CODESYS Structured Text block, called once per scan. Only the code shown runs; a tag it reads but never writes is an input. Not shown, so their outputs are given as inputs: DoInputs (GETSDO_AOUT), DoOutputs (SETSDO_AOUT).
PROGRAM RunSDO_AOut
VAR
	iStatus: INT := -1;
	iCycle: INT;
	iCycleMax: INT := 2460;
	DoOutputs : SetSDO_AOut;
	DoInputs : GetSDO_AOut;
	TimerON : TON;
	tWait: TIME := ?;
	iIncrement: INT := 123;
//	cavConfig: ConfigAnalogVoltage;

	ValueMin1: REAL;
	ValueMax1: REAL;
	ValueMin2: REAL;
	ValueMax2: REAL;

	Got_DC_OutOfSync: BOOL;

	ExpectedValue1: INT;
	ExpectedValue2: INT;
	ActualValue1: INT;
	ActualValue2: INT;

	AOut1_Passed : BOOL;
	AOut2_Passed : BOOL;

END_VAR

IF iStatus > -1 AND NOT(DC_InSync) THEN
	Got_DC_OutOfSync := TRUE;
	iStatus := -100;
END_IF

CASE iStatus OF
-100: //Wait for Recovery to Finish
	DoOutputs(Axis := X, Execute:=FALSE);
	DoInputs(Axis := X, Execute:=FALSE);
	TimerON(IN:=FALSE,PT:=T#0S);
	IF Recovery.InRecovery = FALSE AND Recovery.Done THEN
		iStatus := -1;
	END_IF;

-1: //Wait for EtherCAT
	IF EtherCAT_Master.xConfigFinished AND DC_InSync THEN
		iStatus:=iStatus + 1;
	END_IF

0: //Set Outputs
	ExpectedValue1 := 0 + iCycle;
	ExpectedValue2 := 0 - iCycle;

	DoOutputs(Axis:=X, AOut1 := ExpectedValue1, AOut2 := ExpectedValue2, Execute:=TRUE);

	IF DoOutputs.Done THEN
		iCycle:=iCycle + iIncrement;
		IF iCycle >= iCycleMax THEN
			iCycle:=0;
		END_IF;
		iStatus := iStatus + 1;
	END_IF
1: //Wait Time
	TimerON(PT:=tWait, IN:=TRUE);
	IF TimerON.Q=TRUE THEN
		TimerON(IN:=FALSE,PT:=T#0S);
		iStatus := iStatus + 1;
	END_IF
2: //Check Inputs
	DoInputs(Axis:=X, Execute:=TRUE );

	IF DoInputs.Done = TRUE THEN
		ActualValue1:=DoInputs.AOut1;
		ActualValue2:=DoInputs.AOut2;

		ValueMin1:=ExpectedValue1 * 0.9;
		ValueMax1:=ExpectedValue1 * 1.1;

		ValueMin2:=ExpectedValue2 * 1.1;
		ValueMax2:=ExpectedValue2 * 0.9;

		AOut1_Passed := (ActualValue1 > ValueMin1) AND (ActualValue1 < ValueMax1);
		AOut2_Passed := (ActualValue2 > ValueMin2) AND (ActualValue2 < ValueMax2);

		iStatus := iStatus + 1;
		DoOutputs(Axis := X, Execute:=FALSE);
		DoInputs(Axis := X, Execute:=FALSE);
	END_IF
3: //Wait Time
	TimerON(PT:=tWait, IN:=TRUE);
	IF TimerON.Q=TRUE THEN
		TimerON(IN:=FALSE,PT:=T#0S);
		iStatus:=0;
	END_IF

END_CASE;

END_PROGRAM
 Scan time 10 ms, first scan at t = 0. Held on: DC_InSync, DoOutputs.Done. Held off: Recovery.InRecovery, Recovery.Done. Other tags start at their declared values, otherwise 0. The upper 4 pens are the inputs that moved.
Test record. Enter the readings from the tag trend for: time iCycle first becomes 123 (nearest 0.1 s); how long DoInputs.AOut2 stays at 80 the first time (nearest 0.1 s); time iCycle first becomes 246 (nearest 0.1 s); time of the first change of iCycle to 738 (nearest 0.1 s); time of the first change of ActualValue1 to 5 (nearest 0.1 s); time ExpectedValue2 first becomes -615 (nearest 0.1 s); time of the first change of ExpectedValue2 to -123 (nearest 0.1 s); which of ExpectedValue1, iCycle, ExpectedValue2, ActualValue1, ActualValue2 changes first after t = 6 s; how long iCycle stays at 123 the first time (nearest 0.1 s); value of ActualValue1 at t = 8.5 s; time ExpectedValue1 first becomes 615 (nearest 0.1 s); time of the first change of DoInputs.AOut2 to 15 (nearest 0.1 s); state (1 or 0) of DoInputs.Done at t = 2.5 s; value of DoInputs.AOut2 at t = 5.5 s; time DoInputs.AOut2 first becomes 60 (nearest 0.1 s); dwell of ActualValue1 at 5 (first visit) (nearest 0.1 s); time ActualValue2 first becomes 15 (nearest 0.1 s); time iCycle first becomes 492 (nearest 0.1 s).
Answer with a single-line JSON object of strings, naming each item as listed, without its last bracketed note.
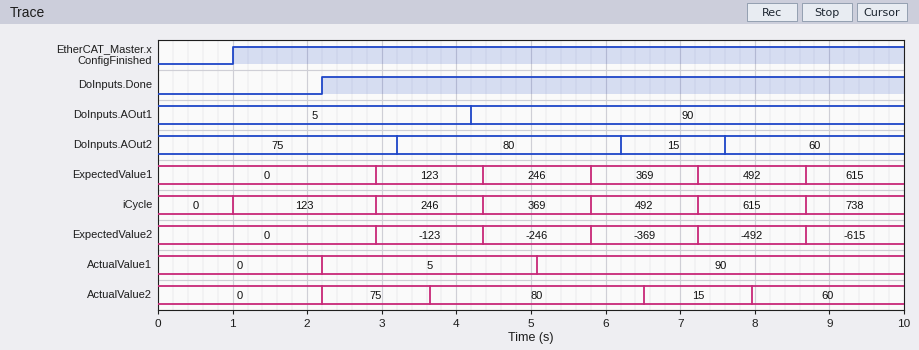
{"time iCycle first becomes 123": "1.0 s", "how long DoInputs.AOut2 stays at 80 the first time": "3.0 s", "time iCycle first becomes 246": "2.9 s", "time of the first change of iCycle to 738": "8.7 s", "time of the first change of ActualValue1 to 5": "2.2 s", "time ExpectedValue2 first becomes -615": "8.7 s", "time of the first change of ExpectedValue2 to -123": "2.9 s", "which of ExpectedValue1, iCycle, ExpectedValue2, ActualValue1, ActualValue2 changes first after t = 6 s": "ActualValue2", "how long iCycle stays at 123 the first time": "1.9 s", "value of ActualValue1 at t = 8.5 s": "90", "time ExpectedValue1 first becomes 615": "8.7 s", "time of the first change of DoInputs.AOut2 to 15": "6.2 s", "state (1 or 0) of DoInputs.Done at t = 2.5 s": "1", "value of DoInputs.AOut2 at t = 5.5 s": "80", "time DoInputs.AOut2 first becomes 60": "7.6 s", "dwell of ActualValue1 at 5 (first visit)": "2.9 s", "time ActualValue2 first becomes 15": "6.5 s", "time iCycle first becomes 492": "5.8 s"}
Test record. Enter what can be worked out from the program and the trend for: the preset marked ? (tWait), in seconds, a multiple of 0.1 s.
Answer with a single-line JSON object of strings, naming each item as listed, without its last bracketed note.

{"the preset marked ? (tWait), in seconds, a multiple of 0.1 s": "0.7 s"}
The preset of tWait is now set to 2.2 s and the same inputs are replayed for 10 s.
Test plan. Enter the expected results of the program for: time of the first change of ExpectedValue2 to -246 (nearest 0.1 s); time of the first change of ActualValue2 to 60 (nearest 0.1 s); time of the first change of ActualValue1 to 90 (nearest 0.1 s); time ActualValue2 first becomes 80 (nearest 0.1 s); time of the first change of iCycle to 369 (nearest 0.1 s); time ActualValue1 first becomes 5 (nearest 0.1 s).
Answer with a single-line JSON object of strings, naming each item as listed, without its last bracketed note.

{"time of the first change of ExpectedValue2 to -246": "9.9 s", "time of the first change of ActualValue2 to 60": "7.7 s", "time of the first change of ActualValue1 to 90": "7.7 s", "time ActualValue2 first becomes 80": "3.2 s", "time of the first change of iCycle to 369": "9.9 s", "time ActualValue1 first becomes 5": "3.2 s"}
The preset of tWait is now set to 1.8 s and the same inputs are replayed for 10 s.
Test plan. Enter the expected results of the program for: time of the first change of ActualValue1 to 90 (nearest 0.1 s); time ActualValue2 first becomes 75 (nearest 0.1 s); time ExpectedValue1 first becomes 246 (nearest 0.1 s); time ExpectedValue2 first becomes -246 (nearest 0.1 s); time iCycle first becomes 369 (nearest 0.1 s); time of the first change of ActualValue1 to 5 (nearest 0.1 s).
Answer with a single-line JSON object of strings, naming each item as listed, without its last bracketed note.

{"time of the first change of ActualValue1 to 90": "6.5 s", "time ActualValue2 first becomes 75": "2.8 s", "time ExpectedValue1 first becomes 246": "8.3 s", "time ExpectedValue2 first becomes -246": "8.3 s", "time iCycle first becomes 369": "8.3 s", "time of the first change of ActualValue1 to 5": "2.8 s"}
